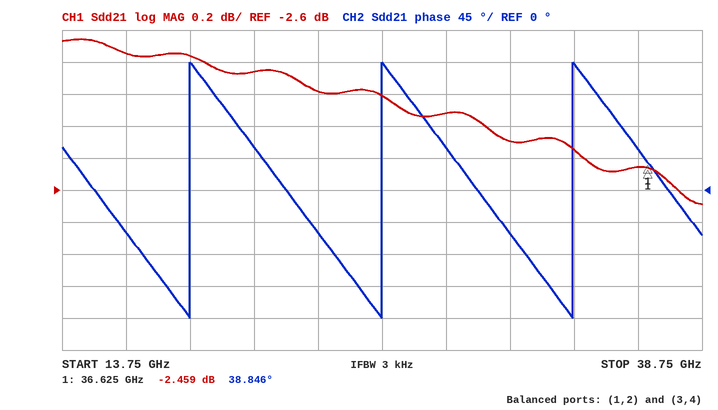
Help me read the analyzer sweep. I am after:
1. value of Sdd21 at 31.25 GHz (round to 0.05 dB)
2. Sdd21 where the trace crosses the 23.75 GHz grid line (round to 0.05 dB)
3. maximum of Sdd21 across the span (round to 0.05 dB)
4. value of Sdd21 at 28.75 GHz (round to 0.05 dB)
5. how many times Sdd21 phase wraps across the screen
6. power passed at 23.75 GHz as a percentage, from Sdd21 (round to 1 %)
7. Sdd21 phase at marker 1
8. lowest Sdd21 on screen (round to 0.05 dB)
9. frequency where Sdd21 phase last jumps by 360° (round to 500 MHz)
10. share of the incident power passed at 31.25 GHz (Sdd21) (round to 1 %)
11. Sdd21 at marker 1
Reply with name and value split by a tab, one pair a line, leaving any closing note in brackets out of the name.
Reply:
value of Sdd21 at 31.25 GHz	-2.30 dB
Sdd21 where the trace crosses the 23.75 GHz grid line	-2.00 dB
maximum of Sdd21 across the span	-1.65 dB
value of Sdd21 at 28.75 GHz	-2.10 dB
how many times Sdd21 phase wraps across the screen	3
power passed at 23.75 GHz as a percentage, from Sdd21	63 %
Sdd21 phase at marker 1	38.846°
lowest Sdd21 on screen	-2.70 dB
frequency where Sdd21 phase last jumps by 360°	33.5 GHz
share of the incident power passed at 31.25 GHz (Sdd21)	59 %
Sdd21 at marker 1	-2.459 dB
